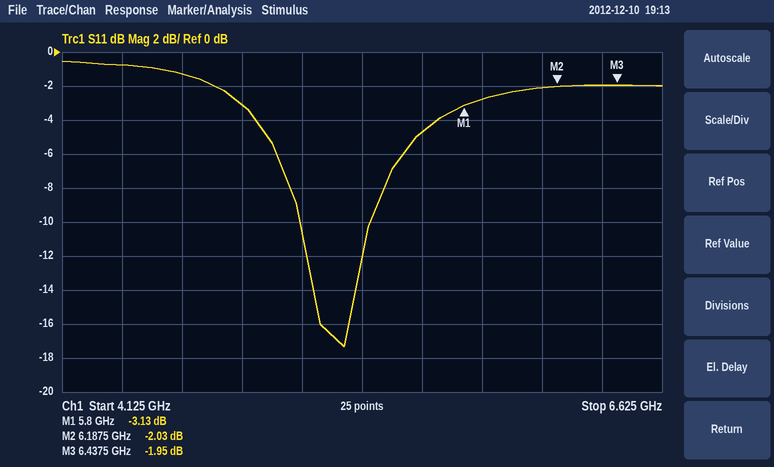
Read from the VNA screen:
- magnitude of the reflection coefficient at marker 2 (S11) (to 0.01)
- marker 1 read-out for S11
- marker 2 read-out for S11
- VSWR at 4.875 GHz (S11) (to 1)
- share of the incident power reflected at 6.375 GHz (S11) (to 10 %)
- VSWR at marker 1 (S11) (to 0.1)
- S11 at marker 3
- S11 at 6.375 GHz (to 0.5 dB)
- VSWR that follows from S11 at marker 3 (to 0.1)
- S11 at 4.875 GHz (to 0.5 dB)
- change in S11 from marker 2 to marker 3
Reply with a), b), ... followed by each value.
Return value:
a) 0.79
b) -3.13 dB
c) -2.03 dB
d) 6
e) 60 %
f) 5.6
g) -1.95 dB
h) -2.0 dB
i) 8.9
j) -3.0 dB
k) 0.08 dB
